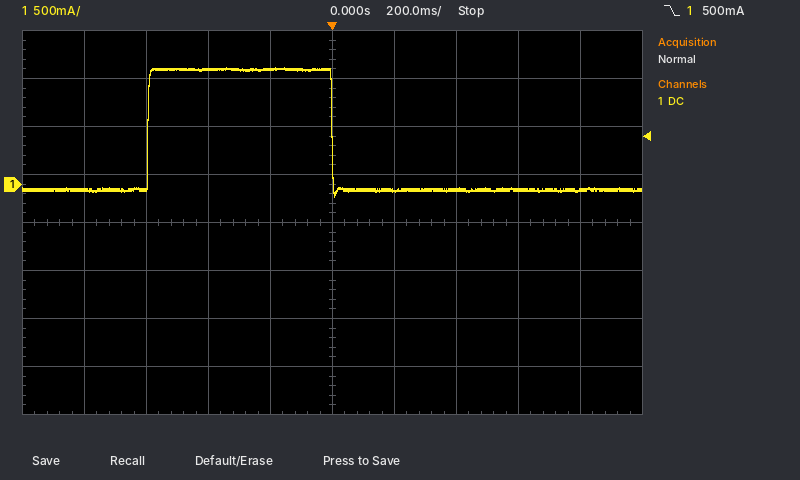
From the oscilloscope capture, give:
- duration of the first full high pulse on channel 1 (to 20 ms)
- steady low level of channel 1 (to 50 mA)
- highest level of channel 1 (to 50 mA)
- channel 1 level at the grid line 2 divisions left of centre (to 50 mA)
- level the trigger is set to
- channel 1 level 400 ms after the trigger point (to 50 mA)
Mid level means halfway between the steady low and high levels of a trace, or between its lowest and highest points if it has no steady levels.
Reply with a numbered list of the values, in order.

1. 600 ms
2. -50 mA
3. 1.20 A
4. 1.20 A
5. 500 mA
6. -50 mA
